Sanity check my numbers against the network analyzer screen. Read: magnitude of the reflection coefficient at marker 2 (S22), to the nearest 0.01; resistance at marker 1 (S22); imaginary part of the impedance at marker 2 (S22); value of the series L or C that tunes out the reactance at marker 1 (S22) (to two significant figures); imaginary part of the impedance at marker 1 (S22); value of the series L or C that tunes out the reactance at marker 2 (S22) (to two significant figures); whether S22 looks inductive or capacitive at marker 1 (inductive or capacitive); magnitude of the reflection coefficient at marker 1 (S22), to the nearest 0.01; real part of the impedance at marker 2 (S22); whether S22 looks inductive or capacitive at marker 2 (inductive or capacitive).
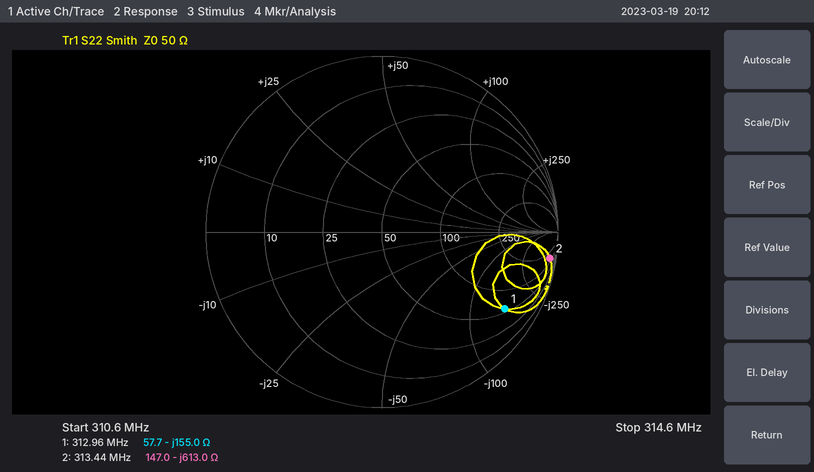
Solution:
0.96
57.7 Ω
-613.0 Ω
79 nH
-155.0 Ω
310 nH
capacitive
0.82
147.0 Ω
capacitive
